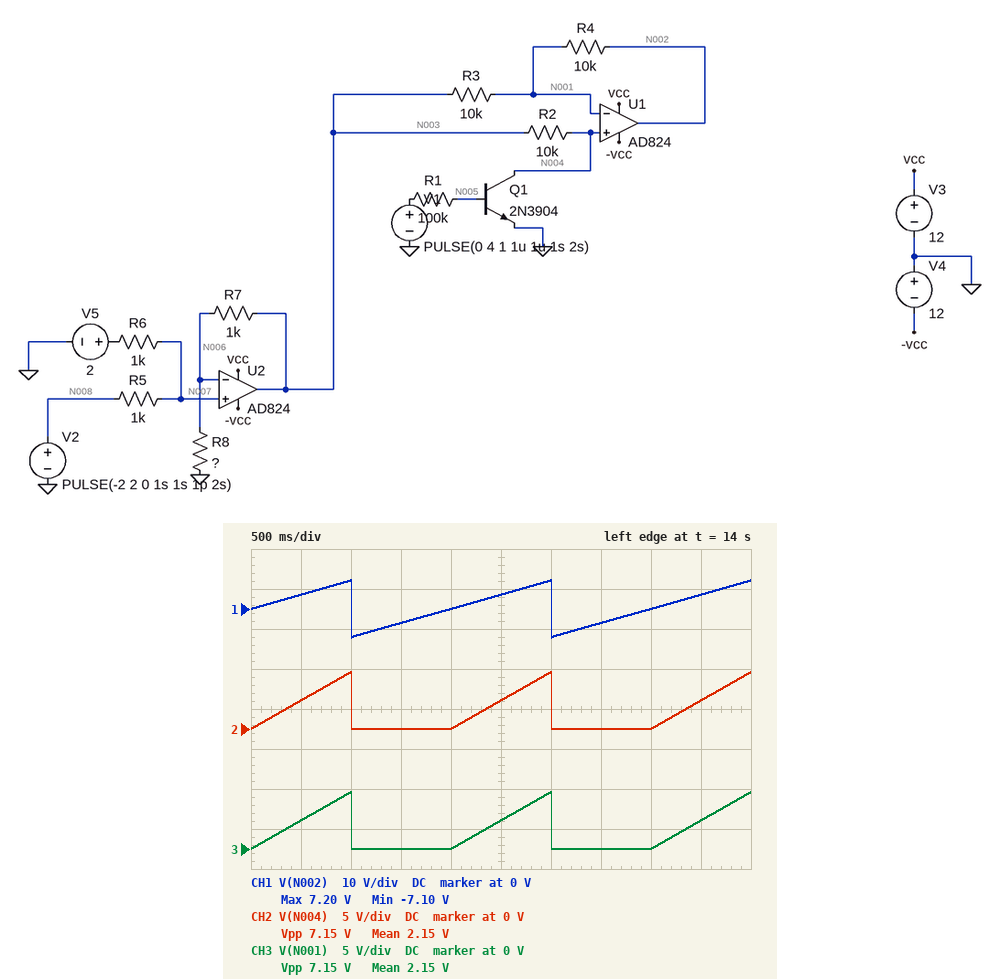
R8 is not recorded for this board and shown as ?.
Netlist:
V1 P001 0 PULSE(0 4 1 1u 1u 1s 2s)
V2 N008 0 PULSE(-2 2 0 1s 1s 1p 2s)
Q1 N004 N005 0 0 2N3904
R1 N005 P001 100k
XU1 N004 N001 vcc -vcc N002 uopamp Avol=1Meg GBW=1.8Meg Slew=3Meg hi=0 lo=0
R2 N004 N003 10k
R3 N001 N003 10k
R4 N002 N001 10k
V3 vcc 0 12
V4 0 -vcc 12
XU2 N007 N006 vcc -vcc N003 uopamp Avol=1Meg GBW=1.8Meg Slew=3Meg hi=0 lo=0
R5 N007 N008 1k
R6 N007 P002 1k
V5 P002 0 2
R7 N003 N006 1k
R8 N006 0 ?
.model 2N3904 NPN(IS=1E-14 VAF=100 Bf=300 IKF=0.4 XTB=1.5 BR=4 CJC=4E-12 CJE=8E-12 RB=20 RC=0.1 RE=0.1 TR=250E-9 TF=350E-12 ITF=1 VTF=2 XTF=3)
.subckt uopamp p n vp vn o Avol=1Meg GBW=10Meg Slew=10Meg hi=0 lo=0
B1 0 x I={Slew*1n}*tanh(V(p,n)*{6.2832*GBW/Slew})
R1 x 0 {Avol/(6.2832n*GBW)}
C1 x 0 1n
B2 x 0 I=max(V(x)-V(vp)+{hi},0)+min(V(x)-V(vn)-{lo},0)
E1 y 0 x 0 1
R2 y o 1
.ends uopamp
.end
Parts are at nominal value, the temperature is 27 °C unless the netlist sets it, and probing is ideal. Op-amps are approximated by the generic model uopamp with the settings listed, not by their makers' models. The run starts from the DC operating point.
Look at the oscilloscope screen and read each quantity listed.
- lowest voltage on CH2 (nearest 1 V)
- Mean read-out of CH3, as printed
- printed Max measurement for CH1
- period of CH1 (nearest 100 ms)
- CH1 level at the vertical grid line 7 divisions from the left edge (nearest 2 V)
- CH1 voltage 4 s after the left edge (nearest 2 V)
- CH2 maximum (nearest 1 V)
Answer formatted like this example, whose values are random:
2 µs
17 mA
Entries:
0 V
2.15 V
7.20 V
2.0 s
-4 V
0 V
7 V
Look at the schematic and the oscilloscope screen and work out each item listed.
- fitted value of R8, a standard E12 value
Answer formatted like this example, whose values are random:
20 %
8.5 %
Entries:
390 Ω
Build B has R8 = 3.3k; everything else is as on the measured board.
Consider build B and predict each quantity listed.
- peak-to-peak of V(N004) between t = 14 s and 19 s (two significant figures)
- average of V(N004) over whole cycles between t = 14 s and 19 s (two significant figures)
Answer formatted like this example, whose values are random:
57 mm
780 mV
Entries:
2.7 V
660 mV
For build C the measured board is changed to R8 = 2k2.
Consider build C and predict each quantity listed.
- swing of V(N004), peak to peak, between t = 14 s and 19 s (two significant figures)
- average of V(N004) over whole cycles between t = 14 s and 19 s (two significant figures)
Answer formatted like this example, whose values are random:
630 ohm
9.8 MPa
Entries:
3.0 V
740 mV
